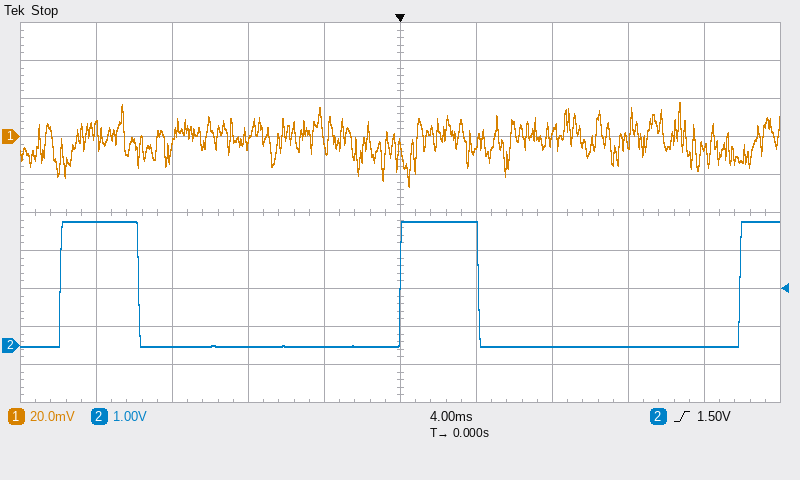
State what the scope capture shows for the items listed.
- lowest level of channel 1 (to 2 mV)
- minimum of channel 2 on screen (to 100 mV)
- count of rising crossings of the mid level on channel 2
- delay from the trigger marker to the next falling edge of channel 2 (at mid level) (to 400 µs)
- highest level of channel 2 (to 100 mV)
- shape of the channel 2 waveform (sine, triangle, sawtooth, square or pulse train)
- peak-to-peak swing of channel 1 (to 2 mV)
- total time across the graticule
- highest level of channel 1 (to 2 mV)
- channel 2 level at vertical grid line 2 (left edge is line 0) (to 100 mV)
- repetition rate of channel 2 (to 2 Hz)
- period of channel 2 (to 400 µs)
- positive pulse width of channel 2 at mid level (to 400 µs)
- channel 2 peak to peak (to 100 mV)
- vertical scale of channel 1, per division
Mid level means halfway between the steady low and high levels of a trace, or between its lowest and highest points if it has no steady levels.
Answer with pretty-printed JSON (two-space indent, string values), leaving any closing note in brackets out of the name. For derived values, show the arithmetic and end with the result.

{
  "lowest level of channel 1": "-26 mV",
  "minimum of channel 2 on screen": "0.0 V",
  "count of rising crossings of the mid level on channel 2": "3",
  "delay from the trigger marker to the next falling edge of channel 2 (at mid level)": "4.0 ms",
  "highest level of channel 2": "3.3 V",
  "shape of the channel 2 waveform": "pulse train",
  "peak-to-peak swing of channel 1": "18 mV − (-26 mV) = 44 mV",
  "total time across the graticule": "40 ms",
  "highest level of channel 1": "18 mV",
  "channel 2 level at vertical grid line 2 (left edge is line 0)": "0.0 V",
  "repetition rate of channel 2": "1 / 18.0 ms ≈ 56 Hz",
  "period of channel 2": "18.0 ms",
  "positive pulse width of channel 2 at mid level": "4.0 ms",
  "channel 2 peak to peak": "3.3 V − (0.0 V) = 3.3 V",
  "vertical scale of channel 1, per division": "20 mV"
}
